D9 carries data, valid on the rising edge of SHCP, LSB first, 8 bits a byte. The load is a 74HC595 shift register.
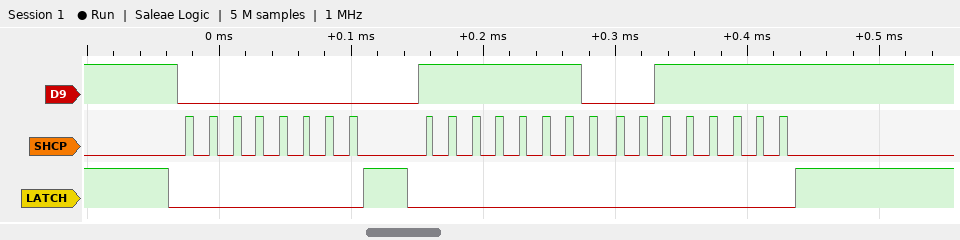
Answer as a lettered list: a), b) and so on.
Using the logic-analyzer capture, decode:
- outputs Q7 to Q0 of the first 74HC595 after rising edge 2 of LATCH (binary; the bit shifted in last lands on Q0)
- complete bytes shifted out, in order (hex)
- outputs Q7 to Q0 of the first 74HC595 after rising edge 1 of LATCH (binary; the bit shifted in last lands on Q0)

a) 00111111
b) 0x00 0x7F 0xFC
c) 00000000
